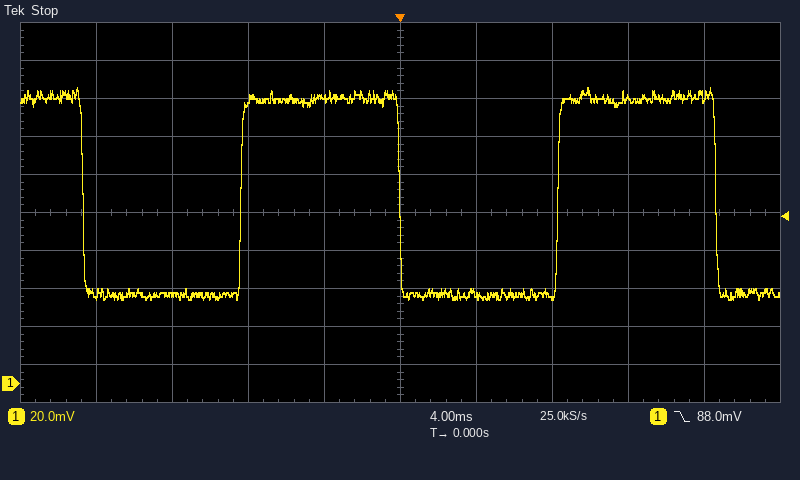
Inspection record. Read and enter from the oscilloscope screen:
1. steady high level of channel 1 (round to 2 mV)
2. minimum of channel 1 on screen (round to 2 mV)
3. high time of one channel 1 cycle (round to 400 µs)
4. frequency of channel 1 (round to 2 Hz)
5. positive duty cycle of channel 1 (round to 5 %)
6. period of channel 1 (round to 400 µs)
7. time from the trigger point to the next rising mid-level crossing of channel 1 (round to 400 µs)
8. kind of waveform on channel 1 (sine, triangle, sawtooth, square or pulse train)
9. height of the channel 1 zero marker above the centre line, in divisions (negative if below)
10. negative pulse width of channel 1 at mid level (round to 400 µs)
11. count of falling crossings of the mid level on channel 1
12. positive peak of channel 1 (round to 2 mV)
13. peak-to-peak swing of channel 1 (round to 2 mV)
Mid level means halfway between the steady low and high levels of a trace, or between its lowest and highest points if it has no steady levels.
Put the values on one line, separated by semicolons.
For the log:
150 mV; 44 mV; 8.4 ms; 60 Hz; 50 %; 16.8 ms; 8.4 ms; square; -4.5 div; 8.4 ms; 3; 156 mV; 112 mV
